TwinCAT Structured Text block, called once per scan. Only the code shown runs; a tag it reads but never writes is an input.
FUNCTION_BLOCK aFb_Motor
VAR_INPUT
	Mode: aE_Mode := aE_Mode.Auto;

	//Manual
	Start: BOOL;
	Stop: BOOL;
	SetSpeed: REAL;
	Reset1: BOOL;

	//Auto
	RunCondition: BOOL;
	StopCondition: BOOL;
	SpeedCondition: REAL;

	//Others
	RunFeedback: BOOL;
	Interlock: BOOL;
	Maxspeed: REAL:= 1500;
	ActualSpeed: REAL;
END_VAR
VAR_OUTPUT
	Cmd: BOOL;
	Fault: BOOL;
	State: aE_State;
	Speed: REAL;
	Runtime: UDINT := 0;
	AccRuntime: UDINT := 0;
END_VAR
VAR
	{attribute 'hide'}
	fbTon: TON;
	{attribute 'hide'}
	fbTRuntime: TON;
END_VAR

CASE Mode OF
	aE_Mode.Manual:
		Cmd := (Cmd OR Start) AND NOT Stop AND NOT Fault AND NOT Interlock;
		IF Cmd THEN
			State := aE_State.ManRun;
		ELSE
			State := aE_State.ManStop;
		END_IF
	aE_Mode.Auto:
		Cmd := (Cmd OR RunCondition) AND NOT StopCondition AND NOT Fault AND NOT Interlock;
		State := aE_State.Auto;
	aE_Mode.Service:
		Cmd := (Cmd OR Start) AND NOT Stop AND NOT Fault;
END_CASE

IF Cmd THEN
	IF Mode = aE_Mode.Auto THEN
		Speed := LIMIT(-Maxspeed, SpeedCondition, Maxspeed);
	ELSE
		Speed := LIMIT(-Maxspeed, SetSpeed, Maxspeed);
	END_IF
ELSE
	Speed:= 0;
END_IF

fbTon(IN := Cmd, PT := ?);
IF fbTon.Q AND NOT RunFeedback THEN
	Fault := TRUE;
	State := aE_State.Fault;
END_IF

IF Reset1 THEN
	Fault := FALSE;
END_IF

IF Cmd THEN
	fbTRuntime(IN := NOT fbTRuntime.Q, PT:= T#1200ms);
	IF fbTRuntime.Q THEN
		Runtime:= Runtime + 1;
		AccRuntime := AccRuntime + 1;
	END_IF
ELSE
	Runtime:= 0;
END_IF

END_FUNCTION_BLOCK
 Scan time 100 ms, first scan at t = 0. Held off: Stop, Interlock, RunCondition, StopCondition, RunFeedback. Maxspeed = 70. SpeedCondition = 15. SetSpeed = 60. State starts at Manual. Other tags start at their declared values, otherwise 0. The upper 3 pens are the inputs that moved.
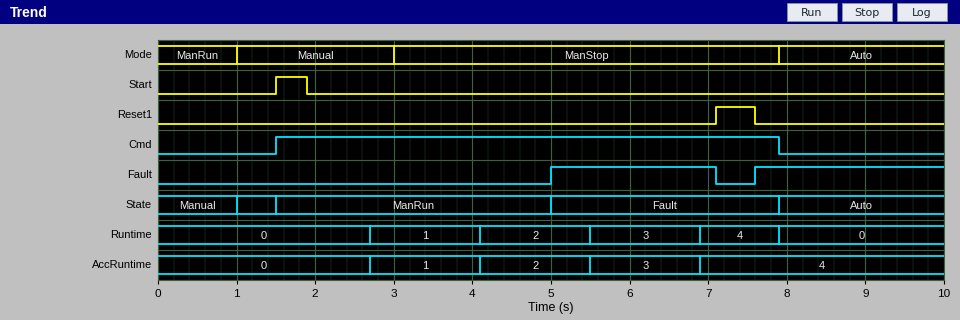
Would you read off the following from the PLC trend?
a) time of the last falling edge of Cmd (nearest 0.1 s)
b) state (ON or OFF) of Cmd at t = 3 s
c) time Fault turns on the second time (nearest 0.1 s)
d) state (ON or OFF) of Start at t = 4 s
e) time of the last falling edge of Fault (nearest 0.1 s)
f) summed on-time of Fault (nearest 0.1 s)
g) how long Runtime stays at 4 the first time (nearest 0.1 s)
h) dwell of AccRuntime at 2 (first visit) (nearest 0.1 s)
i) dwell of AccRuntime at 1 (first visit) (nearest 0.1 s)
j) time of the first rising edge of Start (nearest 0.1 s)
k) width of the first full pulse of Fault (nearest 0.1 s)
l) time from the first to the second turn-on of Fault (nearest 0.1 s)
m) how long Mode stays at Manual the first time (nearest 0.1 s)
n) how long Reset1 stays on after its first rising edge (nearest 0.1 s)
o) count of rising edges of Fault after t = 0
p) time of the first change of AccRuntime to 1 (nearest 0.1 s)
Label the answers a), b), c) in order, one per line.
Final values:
a) 7.9 s
b) ON
c) 7.6 s
d) OFF
e) 7.1 s
f) 4.5 s
g) 1.0 s
h) 1.4 s
i) 1.4 s
j) 1.5 s
k) 2.1 s
l) 2.6 s
m) 2.0 s
n) 0.5 s
o) 2
p) 2.7 s
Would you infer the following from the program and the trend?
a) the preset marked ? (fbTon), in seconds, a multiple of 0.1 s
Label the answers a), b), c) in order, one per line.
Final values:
a) 3.5 s
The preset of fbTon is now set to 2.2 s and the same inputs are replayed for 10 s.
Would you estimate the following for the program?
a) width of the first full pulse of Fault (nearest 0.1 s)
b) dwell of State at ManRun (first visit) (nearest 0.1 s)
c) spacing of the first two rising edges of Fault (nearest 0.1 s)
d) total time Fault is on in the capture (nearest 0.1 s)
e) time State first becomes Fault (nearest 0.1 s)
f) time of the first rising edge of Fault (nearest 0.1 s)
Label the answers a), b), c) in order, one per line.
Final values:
a) 3.4 s
b) 2.2 s
c) 3.9 s
d) 5.8 s
e) 3.7 s
f) 3.7 s
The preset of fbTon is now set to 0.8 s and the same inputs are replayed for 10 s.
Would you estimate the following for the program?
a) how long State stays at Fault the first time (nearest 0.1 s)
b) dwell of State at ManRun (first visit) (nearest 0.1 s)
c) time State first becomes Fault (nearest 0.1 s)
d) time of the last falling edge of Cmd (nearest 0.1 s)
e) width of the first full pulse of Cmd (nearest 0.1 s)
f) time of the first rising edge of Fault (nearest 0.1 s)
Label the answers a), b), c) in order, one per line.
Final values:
a) 0.1 s
b) 0.8 s
c) 2.3 s
d) 2.4 s
e) 0.9 s
f) 2.3 s
